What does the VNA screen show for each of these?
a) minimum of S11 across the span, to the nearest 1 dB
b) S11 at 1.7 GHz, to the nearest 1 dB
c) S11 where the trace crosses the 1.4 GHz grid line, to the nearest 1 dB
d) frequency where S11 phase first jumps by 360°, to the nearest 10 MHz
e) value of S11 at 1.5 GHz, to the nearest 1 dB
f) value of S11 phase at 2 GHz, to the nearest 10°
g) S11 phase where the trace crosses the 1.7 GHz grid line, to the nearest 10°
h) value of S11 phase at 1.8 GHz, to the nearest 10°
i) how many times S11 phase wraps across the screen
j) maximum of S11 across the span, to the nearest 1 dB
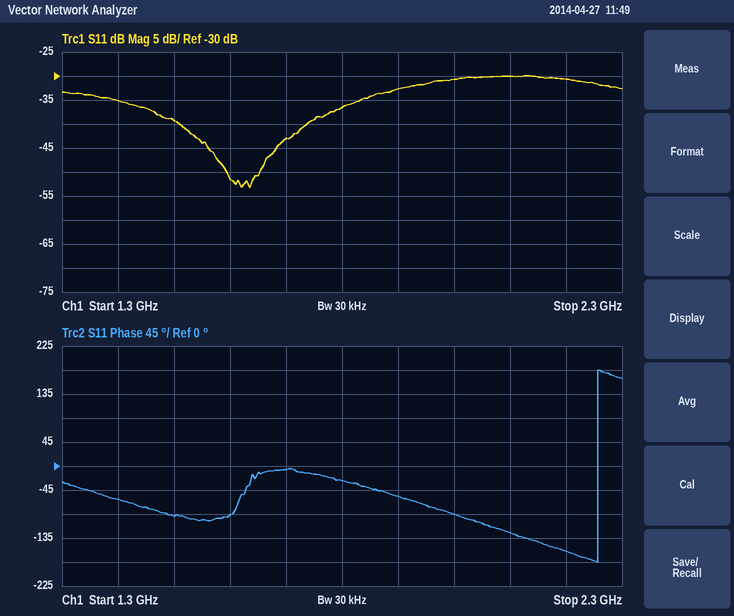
-53 dB
-43 dB
-35 dB
2.26 GHz
-39 dB
-90°
-10°
-30°
1
-30 dB
